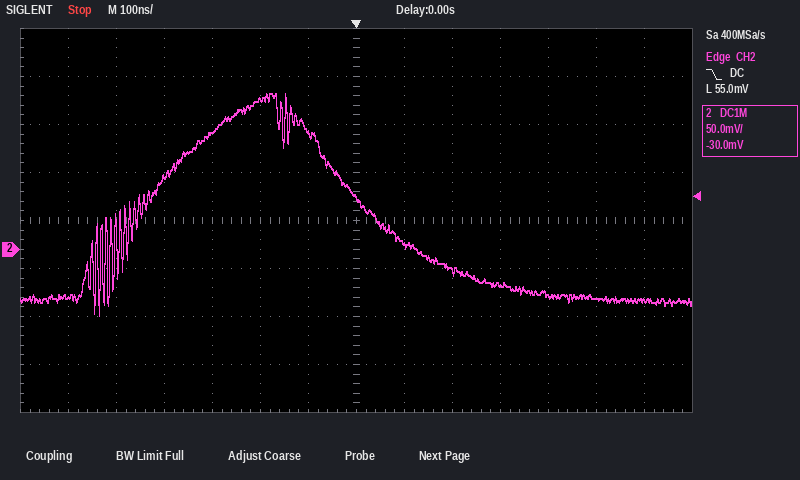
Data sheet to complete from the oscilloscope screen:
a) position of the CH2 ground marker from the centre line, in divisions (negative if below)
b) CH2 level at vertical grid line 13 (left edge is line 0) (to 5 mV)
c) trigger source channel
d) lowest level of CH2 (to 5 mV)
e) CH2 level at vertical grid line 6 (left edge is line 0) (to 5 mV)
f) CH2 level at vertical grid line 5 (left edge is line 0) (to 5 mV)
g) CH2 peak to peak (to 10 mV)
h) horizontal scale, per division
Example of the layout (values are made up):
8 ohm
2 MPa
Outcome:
-0.6 div
-55 mV
CH2
-70 mV
120 mV
155 mV
230 mV
100 ns
